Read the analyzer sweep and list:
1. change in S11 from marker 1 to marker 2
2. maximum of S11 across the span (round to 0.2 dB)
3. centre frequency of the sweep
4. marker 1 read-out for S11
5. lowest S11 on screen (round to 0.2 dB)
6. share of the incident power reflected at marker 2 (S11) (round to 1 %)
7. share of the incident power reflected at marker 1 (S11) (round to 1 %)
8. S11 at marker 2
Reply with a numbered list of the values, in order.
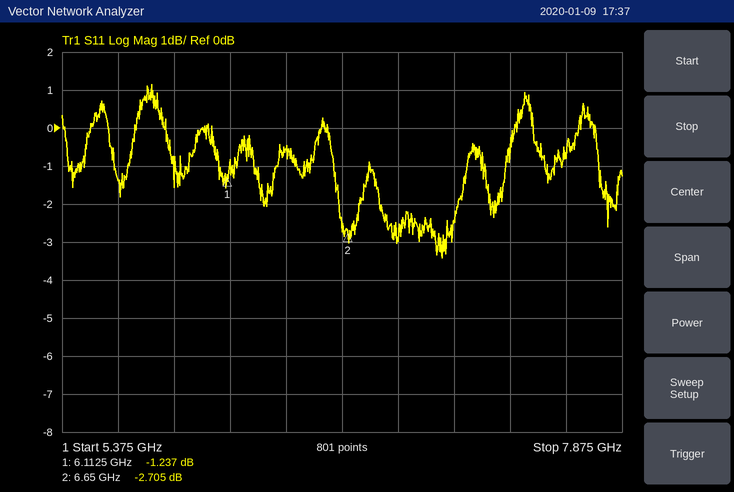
1. -1.468 dB
2. 1.2 dB
3. 6.625 GHz
4. -1.237 dB
5. -3.4 dB
6. 54 %
7. 75 %
8. -2.705 dB
